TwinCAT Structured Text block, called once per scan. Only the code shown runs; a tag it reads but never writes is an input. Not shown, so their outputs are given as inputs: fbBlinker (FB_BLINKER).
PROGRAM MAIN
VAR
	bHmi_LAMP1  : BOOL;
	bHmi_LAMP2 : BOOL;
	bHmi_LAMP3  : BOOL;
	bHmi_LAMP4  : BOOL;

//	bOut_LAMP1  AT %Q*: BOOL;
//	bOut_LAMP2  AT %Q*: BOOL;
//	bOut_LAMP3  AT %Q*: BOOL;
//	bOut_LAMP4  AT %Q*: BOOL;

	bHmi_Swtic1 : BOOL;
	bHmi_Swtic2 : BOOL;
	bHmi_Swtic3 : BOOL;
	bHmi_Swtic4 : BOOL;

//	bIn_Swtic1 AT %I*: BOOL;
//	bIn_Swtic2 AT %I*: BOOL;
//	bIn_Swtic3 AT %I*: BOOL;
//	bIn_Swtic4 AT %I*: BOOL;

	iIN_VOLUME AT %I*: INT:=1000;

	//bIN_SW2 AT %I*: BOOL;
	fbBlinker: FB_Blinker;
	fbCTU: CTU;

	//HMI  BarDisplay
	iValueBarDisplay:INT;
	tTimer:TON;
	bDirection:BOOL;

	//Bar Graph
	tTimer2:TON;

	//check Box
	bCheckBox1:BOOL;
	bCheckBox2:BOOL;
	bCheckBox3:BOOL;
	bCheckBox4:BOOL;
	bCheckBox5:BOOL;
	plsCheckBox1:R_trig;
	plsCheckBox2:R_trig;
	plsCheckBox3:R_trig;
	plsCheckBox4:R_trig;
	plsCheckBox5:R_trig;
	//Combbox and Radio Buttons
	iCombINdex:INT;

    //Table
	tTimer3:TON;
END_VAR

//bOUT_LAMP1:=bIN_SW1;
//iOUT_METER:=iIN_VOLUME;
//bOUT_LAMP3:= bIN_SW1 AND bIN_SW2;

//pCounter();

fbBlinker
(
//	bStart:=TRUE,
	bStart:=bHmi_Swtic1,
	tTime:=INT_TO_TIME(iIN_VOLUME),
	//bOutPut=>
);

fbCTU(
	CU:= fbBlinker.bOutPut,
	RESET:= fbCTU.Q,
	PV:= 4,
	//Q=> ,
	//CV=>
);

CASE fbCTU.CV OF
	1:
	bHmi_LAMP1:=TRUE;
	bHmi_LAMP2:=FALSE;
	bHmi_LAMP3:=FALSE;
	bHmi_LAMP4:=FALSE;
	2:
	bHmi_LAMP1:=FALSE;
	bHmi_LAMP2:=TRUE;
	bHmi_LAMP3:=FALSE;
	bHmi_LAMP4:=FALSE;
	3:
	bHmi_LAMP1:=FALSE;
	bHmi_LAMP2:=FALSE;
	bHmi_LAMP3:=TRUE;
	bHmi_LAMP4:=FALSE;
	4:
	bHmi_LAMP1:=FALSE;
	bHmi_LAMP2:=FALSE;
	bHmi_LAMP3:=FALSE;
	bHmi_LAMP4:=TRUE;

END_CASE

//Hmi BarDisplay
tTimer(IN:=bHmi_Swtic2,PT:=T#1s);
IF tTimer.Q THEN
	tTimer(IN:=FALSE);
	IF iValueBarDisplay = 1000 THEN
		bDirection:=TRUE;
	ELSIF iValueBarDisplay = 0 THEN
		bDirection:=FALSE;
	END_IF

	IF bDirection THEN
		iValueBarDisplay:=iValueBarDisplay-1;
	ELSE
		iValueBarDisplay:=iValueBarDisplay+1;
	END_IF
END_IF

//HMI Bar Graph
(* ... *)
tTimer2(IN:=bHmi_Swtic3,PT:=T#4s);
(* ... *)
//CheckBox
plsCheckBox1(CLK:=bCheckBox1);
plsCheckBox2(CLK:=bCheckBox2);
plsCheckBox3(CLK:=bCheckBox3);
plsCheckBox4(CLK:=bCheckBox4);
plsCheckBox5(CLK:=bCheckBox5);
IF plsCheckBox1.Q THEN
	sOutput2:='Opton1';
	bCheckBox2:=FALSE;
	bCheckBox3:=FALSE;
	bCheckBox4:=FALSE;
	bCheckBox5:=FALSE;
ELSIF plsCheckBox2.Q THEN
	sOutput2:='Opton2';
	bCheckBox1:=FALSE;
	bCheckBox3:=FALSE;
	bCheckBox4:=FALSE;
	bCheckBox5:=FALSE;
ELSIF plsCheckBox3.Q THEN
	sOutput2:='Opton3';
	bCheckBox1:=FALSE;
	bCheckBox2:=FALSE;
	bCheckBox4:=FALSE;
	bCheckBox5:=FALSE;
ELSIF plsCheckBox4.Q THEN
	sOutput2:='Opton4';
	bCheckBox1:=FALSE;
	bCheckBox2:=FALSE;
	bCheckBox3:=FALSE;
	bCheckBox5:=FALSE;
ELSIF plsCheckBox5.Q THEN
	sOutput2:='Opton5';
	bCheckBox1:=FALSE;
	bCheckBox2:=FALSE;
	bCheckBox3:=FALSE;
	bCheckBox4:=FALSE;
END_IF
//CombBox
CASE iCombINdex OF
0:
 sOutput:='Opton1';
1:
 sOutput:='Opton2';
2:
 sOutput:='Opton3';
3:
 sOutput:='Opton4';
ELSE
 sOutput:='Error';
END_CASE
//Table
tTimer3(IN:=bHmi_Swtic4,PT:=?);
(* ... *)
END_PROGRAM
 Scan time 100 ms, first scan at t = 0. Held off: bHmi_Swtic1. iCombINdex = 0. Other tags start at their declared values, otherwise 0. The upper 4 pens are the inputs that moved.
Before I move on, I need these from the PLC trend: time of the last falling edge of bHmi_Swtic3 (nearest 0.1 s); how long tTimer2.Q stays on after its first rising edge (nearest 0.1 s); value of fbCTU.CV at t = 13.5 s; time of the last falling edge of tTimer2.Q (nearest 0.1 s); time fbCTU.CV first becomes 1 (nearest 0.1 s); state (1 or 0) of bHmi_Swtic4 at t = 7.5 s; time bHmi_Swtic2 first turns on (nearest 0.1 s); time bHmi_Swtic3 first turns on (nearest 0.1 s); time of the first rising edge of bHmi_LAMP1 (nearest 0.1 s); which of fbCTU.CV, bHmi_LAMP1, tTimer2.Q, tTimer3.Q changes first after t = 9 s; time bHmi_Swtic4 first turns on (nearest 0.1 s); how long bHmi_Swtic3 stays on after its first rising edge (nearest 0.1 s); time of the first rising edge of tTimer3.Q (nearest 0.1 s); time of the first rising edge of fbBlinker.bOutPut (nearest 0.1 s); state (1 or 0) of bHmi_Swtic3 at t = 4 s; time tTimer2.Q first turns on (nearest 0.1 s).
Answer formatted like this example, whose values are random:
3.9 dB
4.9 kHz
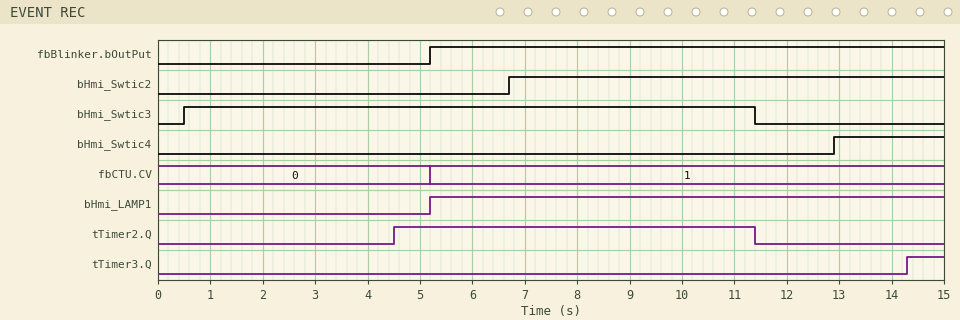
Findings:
11.4 s
6.9 s
1
11.4 s
5.2 s
0
6.7 s
0.5 s
5.2 s
tTimer2.Q
12.9 s
10.9 s
14.3 s
5.2 s
1
4.5 s
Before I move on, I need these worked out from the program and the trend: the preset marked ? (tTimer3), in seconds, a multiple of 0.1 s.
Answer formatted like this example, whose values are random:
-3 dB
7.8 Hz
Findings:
1.4 s
